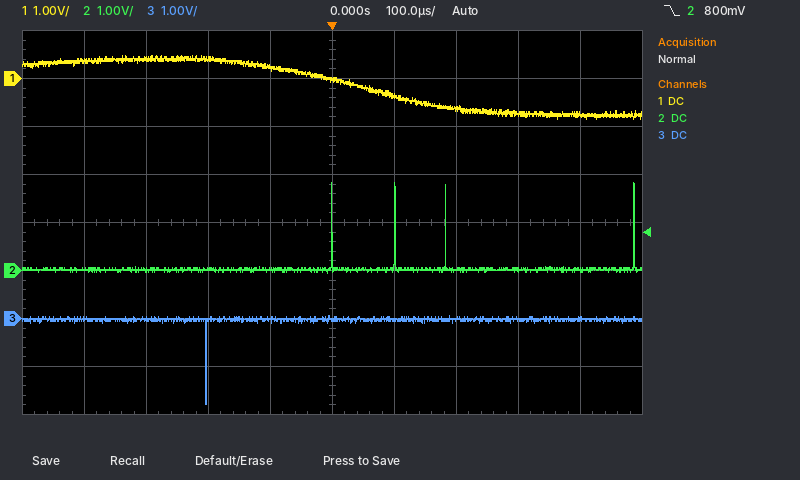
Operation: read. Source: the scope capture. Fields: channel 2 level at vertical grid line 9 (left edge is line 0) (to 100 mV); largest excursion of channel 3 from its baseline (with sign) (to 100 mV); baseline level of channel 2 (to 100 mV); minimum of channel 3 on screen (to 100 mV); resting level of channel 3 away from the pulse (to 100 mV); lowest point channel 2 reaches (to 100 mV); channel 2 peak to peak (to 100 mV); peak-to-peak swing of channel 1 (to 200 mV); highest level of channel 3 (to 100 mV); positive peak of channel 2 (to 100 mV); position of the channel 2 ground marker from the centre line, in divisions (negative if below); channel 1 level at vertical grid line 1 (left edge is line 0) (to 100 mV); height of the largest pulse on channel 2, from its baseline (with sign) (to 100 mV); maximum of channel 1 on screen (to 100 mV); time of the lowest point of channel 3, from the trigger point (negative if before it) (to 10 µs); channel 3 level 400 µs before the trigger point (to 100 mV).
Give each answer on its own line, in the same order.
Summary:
0.0 V
-1.8 V
0.0 V
-1.8 V
0.0 V
-100 mV
1.9 V
1.4 V
100 mV
1.8 V
-1.0 div
400 mV
+1.8 V
500 mV
-200 µs
0.0 V
